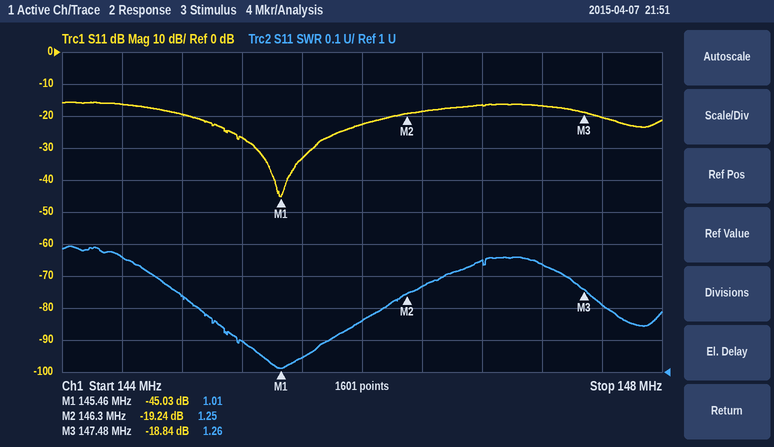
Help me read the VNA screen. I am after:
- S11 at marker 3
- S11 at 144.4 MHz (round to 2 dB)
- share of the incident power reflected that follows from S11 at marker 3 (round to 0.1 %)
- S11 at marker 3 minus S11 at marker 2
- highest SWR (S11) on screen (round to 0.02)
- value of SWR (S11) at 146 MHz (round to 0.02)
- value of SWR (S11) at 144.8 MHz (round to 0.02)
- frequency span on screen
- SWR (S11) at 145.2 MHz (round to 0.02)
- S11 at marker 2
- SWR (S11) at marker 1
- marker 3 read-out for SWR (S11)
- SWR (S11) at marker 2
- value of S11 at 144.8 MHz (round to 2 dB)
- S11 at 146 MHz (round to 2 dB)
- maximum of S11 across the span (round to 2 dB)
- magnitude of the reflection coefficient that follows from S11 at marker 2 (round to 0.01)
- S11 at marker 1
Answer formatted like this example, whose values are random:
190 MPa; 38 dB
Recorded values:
-18.84 dB; -16 dB; 1.3 %; 0.40 dB; 1.40; 1.16; 1.24; 4 MHz; 1.10; -19.24 dB; 1.01; 1.26; 1.25; -20 dB; -22 dB; -16 dB; 0.11; -45.03 dB
